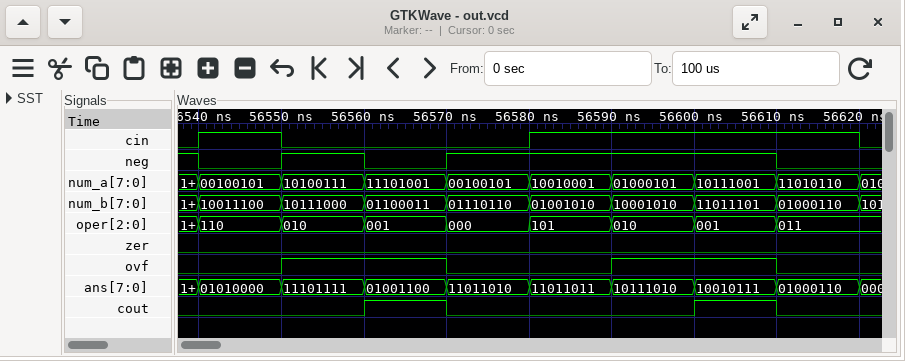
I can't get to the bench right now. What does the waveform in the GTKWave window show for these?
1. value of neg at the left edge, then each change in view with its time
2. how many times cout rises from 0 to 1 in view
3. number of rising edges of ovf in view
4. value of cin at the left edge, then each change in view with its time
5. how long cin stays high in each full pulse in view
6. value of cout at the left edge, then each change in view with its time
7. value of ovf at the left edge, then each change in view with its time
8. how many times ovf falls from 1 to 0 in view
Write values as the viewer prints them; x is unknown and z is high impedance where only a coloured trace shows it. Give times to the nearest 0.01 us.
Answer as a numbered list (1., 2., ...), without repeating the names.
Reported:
1. 1, 0 at 56.54 us, 1 at 56.55 us, 0 at 56.56 us, 1 at 56.57 us, 0 at 56.61 us
2. 2
3. 2
4. 0, 1 at 56.54 us, 0 at 56.55 us, 1 at 56.58 us, 0 at 56.62 us
5. 0.01 us, 0.04 us
6. 0, 1 at 56.56 us, 0 at 56.57 us, 1 at 56.6 us, 0 at 56.61 us
7. 0, 1 at 56.55 us, 0 at 56.57 us, 1 at 56.59 us, 0 at 56.61 us
8. 2
